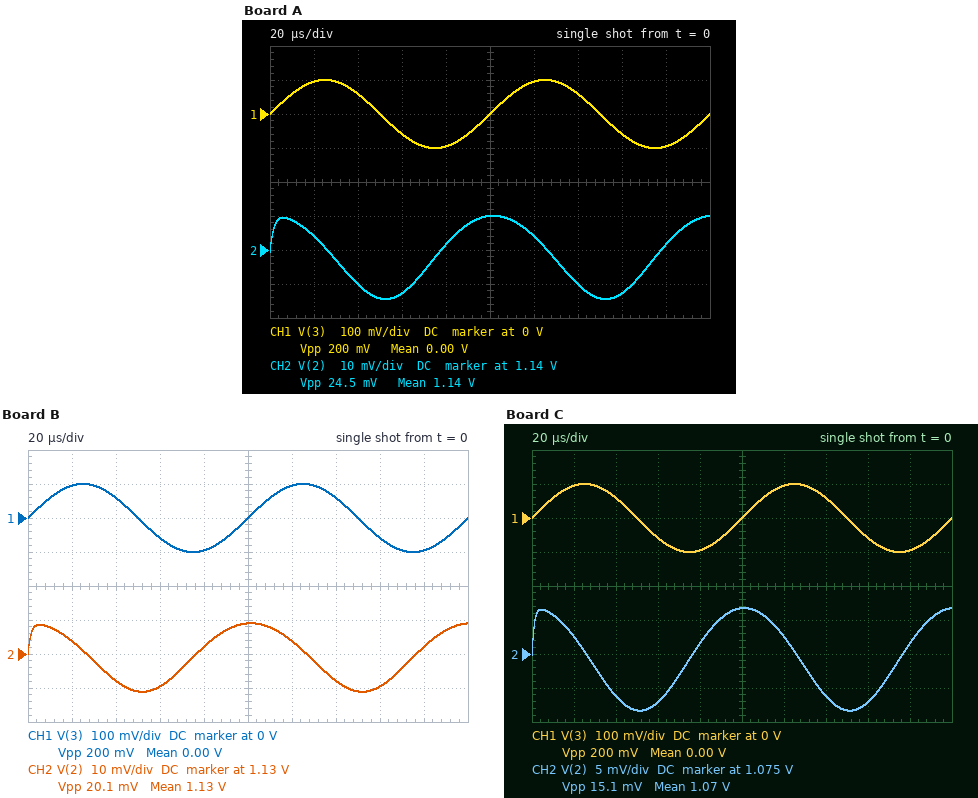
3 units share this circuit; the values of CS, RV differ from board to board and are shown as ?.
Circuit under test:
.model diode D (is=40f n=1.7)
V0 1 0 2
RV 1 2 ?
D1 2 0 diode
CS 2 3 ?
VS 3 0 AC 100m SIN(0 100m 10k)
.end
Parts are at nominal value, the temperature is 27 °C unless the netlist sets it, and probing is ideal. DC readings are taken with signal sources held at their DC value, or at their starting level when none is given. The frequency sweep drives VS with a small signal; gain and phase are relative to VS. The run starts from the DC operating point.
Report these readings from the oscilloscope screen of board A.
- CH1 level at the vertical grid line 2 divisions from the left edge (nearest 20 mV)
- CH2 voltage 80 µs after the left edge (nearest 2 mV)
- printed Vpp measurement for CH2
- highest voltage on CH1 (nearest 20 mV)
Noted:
60 mV
1.142 V
24.5 mV
100 mV
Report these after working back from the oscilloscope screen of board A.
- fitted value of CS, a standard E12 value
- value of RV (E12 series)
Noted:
330 nF
120 Ω
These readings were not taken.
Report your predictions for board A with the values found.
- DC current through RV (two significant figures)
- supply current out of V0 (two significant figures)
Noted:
7.2 mA
7.2 mA
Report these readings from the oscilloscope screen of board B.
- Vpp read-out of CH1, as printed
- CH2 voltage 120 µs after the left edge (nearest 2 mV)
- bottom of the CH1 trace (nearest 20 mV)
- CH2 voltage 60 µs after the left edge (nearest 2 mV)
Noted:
200 mV
1.134 V
-100 mV
1.120 V
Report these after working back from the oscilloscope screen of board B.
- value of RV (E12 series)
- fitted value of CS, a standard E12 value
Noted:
150 Ω
220 nF
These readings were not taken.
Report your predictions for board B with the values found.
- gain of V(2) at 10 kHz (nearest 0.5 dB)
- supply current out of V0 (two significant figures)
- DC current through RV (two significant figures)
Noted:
-20.0 dB
5.8 mA
5.8 mA
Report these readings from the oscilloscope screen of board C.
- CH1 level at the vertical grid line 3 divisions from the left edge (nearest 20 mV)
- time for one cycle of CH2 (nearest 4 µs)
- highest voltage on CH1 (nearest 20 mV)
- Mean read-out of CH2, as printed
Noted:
-60 mV
100 µs
100 mV
1.07 V
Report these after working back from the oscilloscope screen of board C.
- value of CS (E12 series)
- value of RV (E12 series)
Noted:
47 nF
560 Ω
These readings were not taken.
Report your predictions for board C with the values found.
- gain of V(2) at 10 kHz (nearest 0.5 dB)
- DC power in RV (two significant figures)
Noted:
-22.5 dB
1.5 mW
